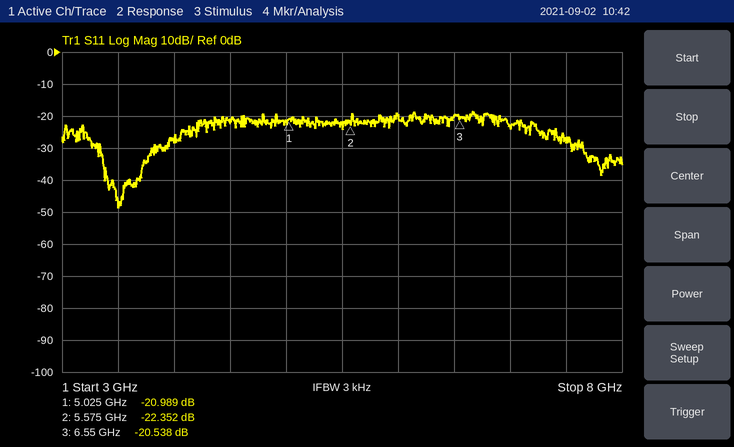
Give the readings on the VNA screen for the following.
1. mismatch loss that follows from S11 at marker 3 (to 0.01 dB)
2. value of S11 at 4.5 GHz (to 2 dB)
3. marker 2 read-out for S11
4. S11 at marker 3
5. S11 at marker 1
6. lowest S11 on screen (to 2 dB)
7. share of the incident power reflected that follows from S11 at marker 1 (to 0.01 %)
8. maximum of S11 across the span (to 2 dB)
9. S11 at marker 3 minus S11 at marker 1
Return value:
0.04 dB
-22 dB
-22.352 dB
-20.538 dB
-20.989 dB
-48 dB
0.80 %
-18 dB
0.451 dB
